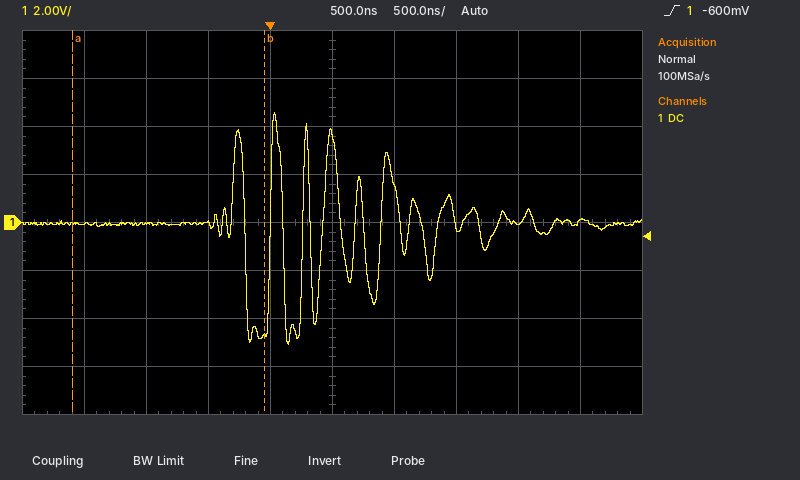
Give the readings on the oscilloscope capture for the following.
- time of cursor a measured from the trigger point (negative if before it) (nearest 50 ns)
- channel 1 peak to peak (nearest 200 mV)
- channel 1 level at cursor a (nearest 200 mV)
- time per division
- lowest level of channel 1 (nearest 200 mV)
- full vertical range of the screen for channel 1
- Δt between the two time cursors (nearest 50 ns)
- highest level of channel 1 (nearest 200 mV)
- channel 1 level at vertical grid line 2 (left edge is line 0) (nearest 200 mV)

-1.60 µs
9.6 V
0.0 V
500 ns
-5.0 V
16 V
1.55 µs
4.6 V
0.0 V
